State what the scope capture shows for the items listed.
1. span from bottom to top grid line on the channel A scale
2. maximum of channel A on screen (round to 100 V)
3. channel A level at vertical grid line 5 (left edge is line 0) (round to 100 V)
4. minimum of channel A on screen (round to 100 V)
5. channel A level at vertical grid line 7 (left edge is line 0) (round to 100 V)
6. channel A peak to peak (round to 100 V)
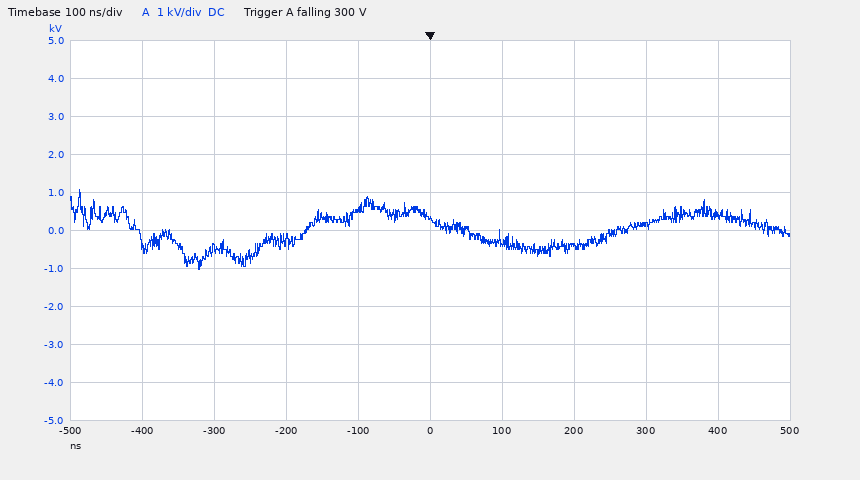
10 kV
1.1 kV
300 V
-1.0 kV
-400 V
2.1 kV
